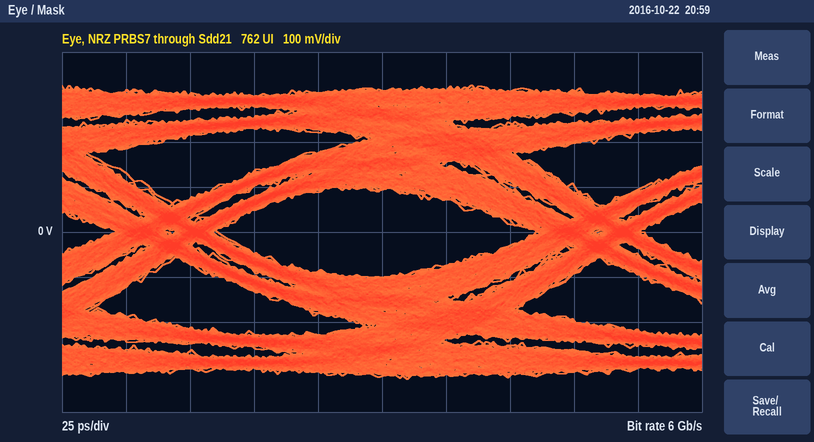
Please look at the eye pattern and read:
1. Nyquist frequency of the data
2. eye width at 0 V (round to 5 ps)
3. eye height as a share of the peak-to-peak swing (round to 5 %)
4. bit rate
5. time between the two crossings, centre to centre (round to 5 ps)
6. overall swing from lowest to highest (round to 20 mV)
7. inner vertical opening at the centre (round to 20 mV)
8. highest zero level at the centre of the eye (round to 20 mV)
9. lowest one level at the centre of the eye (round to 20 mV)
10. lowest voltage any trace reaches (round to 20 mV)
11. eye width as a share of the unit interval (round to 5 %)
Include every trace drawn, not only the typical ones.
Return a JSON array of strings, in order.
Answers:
["3 GHz", "125 ps", "30 %", "6 Gb/s", "165 ps", "660 mV", "200 mV", "-100 mV", "100 mV", "-320 mV", "75 %"]
